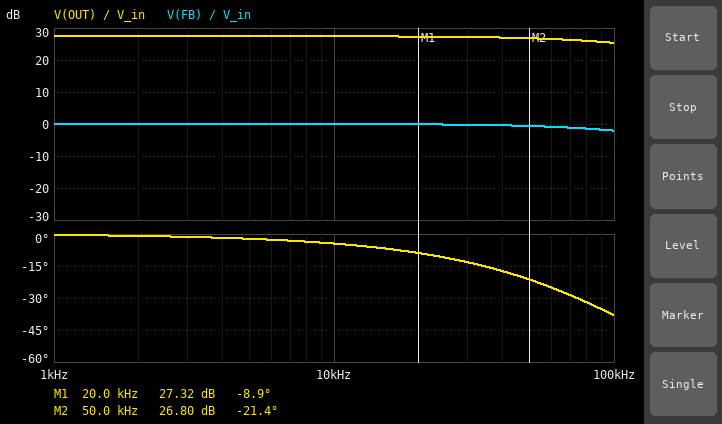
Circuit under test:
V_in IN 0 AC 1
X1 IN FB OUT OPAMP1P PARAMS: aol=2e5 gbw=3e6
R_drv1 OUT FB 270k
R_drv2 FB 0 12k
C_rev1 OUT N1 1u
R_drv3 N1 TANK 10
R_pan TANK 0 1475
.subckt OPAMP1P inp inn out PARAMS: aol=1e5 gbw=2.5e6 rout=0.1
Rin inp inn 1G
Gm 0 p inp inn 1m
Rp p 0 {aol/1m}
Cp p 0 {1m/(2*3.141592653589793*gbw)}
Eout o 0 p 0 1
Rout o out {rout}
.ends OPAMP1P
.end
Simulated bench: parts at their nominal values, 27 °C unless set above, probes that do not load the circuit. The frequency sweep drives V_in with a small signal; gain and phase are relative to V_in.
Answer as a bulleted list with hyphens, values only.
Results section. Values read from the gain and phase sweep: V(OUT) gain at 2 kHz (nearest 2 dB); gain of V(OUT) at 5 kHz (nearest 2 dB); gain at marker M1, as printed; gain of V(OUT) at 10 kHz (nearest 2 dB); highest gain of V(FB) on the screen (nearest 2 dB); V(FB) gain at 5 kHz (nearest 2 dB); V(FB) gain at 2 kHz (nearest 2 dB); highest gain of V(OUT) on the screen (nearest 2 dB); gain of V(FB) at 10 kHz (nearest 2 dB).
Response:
- 28 dB
- 28 dB
- 27.32 dB
- 28 dB
- 0 dB
- 0 dB
- 0 dB
- 28 dB
- 0 dB
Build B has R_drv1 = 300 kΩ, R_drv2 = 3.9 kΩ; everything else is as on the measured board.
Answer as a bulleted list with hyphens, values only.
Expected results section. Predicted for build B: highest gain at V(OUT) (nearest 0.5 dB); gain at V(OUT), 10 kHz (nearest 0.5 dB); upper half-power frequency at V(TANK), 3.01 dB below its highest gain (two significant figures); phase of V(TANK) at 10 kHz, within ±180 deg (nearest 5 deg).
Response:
- 38.0 dB
- 37.5 dB
- 39 kHz
- -15 deg
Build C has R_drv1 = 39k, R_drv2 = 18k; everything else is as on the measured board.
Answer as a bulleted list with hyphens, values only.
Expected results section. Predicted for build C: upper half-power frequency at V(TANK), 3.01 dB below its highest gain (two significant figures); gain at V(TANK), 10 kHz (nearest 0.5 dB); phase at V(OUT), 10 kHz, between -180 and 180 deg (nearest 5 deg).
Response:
- 950 kHz
- 10.0 dB
- 0 deg
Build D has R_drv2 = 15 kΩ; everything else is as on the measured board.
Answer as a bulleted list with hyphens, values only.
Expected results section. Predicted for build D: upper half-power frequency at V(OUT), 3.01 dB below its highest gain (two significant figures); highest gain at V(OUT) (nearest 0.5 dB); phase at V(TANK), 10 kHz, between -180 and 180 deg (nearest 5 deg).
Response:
- 160 kHz
- 25.5 dB
- -5 deg
